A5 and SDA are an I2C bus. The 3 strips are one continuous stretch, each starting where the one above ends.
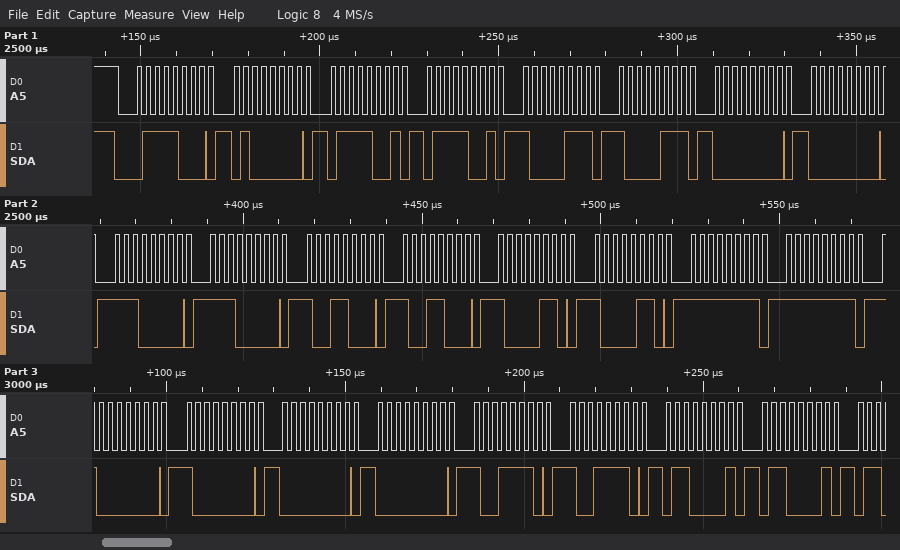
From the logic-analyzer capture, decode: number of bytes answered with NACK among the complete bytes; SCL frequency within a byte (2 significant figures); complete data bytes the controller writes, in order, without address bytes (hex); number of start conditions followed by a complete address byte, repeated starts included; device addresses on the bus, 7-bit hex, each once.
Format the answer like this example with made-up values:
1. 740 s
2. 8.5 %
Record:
1. 0
2. 400 kHz
3. 40 79 79 87 87 00 00 E0 E0 98 98 86 86 FF FF 80 80 00 00 9E 9E 61 61
4. 1
5. 0x3C
